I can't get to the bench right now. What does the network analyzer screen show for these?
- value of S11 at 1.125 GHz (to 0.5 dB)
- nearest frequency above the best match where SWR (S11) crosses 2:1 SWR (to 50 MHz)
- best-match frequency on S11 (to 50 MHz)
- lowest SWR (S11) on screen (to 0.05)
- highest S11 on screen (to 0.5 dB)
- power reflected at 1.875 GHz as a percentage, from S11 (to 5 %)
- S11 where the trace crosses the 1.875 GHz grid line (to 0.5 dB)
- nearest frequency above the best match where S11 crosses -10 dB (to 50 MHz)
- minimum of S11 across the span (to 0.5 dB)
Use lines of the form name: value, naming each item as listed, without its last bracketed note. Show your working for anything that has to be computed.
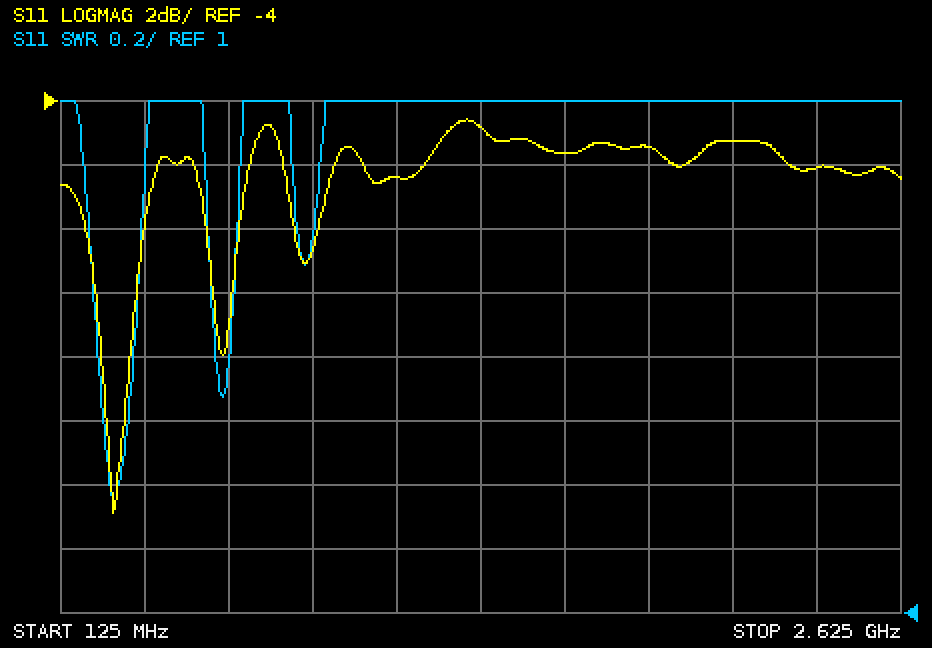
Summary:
value of S11 at 1.125 GHz: -6.5 dB
nearest frequency above the best match where SWR (S11) crosses 2:1 SWR: 350 MHz
best-match frequency on S11: 300 MHz
lowest SWR (S11) on screen: 1.35
highest S11 on screen: -4.5 dB
power reflected at 1.875 GHz as a percentage, from S11: 10^(-5.5/10) ≈ 28.2 %, so 30 % to the nearest 5 %
S11 where the trace crosses the 1.875 GHz grid line: -5.5 dB
nearest frequency above the best match where S11 crosses -10 dB: 350 MHz
minimum of S11 across the span: -17.0 dB
